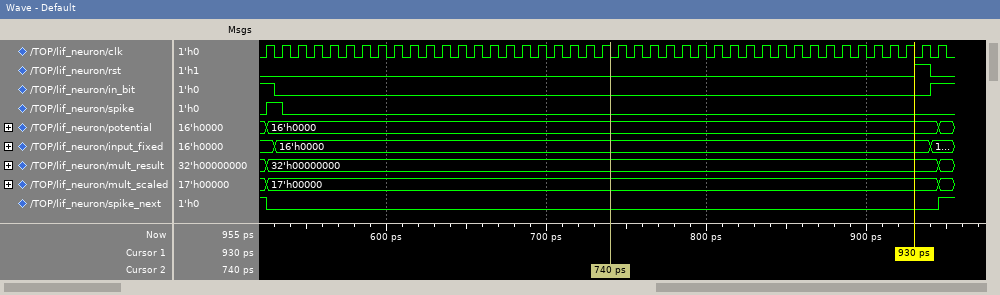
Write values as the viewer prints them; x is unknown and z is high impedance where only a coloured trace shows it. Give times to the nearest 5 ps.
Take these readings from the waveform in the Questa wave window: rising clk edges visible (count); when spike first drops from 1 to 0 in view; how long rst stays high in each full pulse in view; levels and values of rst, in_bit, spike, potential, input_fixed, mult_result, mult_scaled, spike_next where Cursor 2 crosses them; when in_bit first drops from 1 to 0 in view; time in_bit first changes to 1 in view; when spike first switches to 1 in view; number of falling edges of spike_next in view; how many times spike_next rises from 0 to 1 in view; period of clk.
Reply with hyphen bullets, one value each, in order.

- 43
- 535 ps
- 10 ps
- rst=0, in_bit=0, spike=0, potential=16'h0000, input_fixed=16'h0000, mult_result=32'h00000000, mult_scaled=17'h00000, spike_next=0
- 530 ps
- 940 ps
- 525 ps
- 1
- 1
- 10 ps
